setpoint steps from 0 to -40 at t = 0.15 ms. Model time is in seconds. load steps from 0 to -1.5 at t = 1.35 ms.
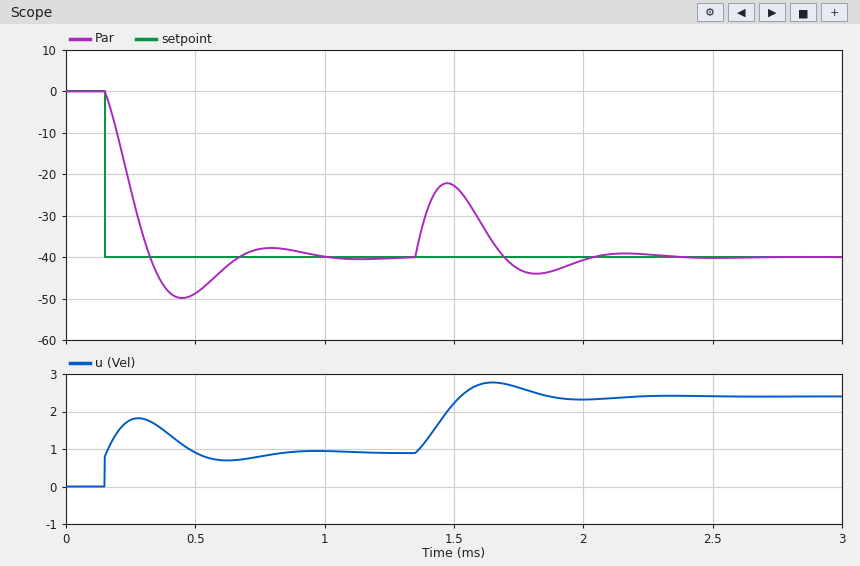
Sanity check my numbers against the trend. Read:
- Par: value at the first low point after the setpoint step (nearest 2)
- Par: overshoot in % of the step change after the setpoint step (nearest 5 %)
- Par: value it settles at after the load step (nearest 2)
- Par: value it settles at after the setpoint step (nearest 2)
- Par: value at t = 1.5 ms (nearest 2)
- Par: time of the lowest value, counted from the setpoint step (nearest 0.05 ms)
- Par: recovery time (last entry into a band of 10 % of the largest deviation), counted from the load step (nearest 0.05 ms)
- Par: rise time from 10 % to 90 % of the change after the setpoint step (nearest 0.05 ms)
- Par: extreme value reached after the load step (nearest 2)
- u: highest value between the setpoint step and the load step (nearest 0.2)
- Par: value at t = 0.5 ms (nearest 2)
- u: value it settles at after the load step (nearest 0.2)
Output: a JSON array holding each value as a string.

["-50", "25 %", "-40", "-40", "-22", "0.30 ms", "0.60 ms", "0.15 ms", "-22", "1.8", "-48", "2.4"]
